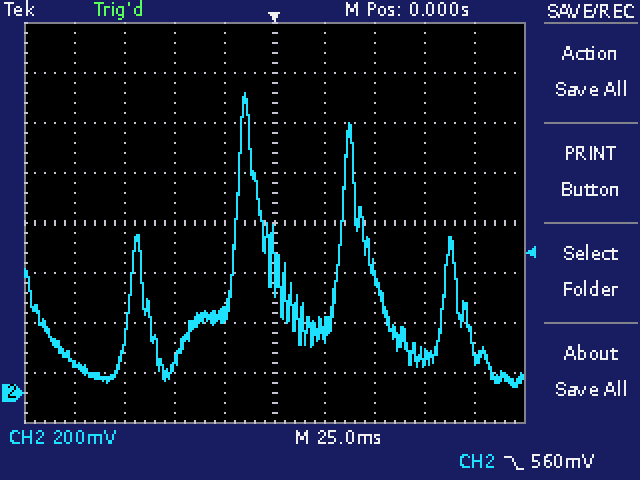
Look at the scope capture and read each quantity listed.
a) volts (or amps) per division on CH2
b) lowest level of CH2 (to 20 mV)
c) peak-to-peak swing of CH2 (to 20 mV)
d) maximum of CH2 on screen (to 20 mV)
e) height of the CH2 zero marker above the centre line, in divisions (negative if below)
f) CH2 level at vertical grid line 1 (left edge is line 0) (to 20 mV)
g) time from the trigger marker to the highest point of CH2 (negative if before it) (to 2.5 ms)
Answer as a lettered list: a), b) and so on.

a) 200 mV
b) 20 mV
c) 1.18 V
d) 1.20 V
e) -3.4 div
f) 120 mV
g) -15.0 ms
